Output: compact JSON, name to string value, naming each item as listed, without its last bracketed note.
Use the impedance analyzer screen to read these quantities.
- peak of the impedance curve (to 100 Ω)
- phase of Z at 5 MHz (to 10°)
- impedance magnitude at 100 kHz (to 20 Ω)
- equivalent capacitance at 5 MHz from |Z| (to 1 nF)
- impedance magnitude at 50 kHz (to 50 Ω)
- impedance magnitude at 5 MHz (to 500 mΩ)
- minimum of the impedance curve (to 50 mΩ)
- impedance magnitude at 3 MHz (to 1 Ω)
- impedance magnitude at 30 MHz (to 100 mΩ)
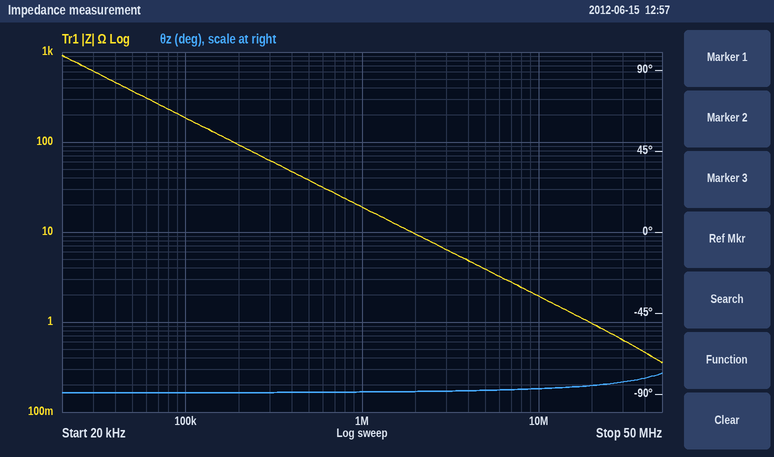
{"peak of the impedance curve": "900 Ω", "phase of Z at 5 MHz": "-90°", "impedance magnitude at 100 kHz": "180 Ω", "equivalent capacitance at 5 MHz from |Z|": "8 nF", "impedance magnitude at 50 kHz": "350 Ω", "impedance magnitude at 5 MHz": "4.0 Ω", "minimum of the impedance curve": "350 mΩ", "impedance magnitude at 3 MHz": "6 Ω", "impedance magnitude at 30 MHz": "600 mΩ"}
